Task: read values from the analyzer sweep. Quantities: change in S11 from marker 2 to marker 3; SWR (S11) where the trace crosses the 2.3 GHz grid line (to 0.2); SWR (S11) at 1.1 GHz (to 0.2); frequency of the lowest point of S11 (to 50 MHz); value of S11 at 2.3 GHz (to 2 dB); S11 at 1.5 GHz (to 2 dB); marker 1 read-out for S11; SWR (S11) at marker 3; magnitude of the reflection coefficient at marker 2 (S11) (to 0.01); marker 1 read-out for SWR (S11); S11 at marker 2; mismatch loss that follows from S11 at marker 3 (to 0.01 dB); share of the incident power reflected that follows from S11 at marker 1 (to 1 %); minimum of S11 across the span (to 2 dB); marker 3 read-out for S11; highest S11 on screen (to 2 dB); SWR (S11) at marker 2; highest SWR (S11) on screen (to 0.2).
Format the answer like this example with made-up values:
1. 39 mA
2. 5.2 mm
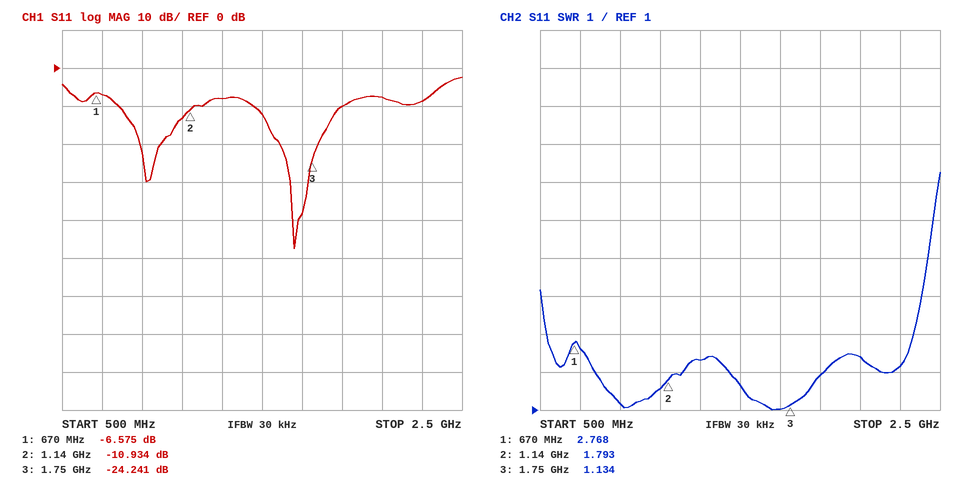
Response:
1. -13.307 dB
2. 2.2
3. 1.6
4. 1.65 GHz
5. -8 dB
6. -12 dB
7. -6.575 dB
8. 1.134
9. 0.28
10. 2.768
11. -10.934 dB
12. 0.02 dB
13. 22 %
14. -48 dB
15. -24.241 dB
16. -2 dB
17. 1.793
18. 7.2
